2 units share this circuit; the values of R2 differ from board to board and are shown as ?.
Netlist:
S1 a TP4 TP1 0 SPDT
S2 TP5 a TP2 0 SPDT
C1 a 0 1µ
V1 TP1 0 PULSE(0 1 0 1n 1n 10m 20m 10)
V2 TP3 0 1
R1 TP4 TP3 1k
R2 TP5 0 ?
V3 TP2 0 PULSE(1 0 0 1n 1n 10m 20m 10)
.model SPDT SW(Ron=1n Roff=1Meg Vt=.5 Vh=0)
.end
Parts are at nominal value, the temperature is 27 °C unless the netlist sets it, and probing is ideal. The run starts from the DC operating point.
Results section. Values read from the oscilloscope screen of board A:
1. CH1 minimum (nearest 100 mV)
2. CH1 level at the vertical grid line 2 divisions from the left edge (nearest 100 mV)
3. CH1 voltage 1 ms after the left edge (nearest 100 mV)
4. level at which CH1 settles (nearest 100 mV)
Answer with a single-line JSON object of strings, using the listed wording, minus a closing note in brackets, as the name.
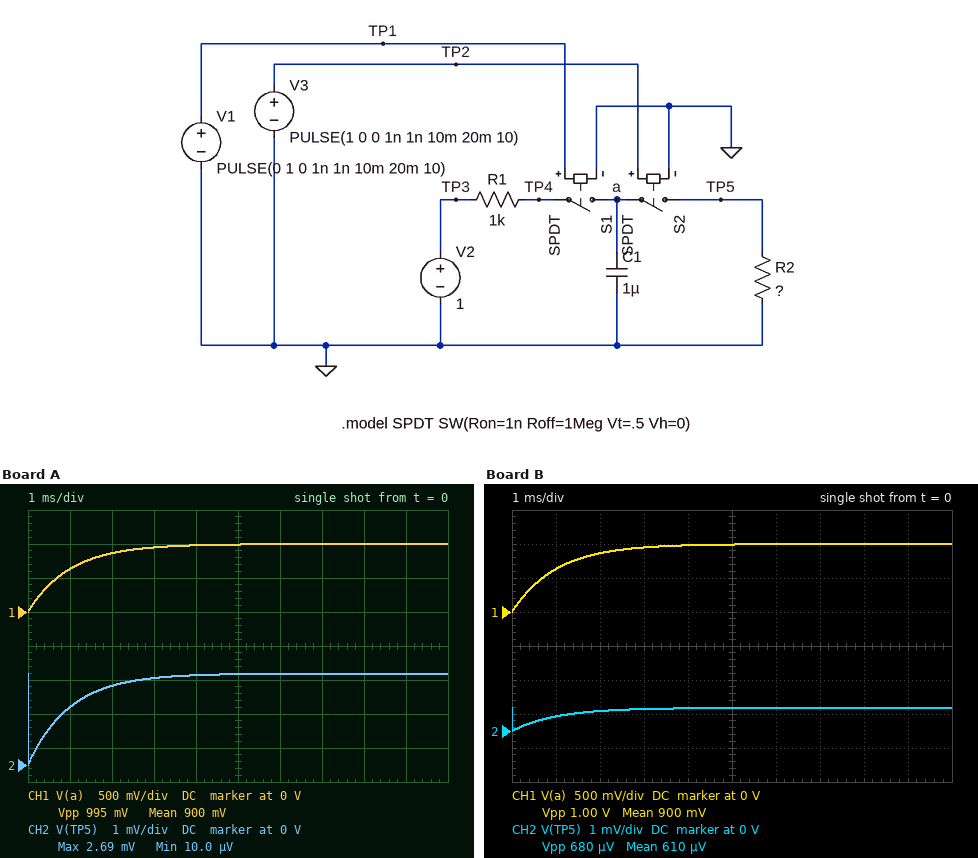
{"CH1 minimum": "0 V", "CH1 level at the vertical grid line 2 divisions from the left edge": "900 mV", "CH1 voltage 1 ms after the left edge": "600 mV", "level at which CH1 settles": "1.0 V"}
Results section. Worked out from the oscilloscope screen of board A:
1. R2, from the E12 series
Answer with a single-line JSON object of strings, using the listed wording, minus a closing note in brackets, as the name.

{"R2, from the E12 series": "2.7 kΩ"}
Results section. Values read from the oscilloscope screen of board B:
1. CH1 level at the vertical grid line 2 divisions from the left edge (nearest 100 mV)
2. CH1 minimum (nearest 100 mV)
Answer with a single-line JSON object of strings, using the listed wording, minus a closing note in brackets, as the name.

{"CH1 level at the vertical grid line 2 divisions from the left edge": "900 mV", "CH1 minimum": "0 V"}
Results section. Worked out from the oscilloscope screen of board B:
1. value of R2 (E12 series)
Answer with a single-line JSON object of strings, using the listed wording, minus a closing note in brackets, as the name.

{"value of R2": "680 Ω"}
